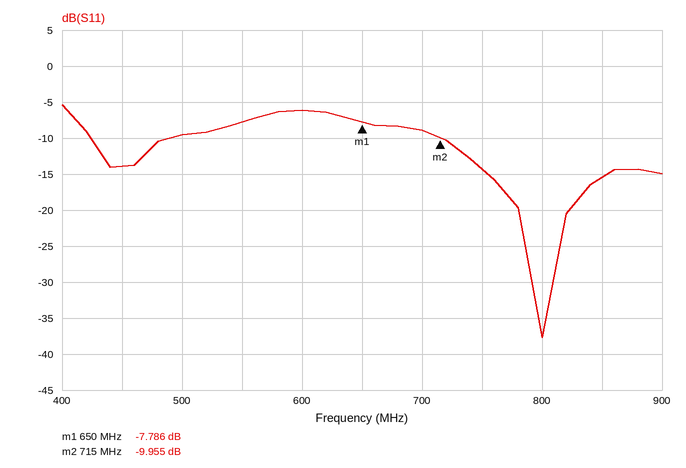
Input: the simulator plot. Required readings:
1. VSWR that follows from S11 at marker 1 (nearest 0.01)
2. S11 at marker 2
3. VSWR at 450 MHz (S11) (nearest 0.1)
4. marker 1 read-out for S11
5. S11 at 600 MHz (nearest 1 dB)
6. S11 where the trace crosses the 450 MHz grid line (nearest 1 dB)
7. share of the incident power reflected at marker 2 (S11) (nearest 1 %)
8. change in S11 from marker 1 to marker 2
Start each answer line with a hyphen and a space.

- 2.38
- -9.955 dB
- 1.5
- -7.786 dB
- -6 dB
- -14 dB
- 10 %
- -2.169 dB
